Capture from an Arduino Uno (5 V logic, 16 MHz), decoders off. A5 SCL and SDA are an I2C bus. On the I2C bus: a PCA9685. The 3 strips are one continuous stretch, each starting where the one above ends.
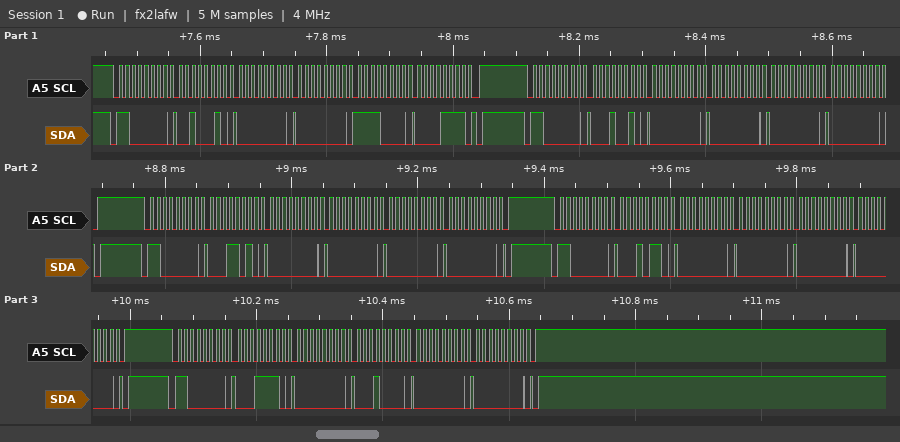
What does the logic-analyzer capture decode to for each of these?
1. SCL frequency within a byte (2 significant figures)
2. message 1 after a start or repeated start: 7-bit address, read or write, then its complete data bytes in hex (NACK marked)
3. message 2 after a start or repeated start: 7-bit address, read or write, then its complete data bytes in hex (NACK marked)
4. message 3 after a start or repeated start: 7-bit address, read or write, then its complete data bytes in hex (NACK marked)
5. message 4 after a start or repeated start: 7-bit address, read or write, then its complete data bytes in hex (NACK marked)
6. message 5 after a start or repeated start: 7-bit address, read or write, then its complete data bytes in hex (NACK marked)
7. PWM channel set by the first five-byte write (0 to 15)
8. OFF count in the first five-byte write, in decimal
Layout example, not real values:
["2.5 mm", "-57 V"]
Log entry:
["100 kHz", "0x60 write: 22 00 00 F0 0F", "0x60 write: 12 00 00 00 00", "0x60 write: 1A 00 00 00 00", "0x60 write: 16 00 00 00 00", "0x60 write: 1E 00 10 00 00", "7", "4080"]
